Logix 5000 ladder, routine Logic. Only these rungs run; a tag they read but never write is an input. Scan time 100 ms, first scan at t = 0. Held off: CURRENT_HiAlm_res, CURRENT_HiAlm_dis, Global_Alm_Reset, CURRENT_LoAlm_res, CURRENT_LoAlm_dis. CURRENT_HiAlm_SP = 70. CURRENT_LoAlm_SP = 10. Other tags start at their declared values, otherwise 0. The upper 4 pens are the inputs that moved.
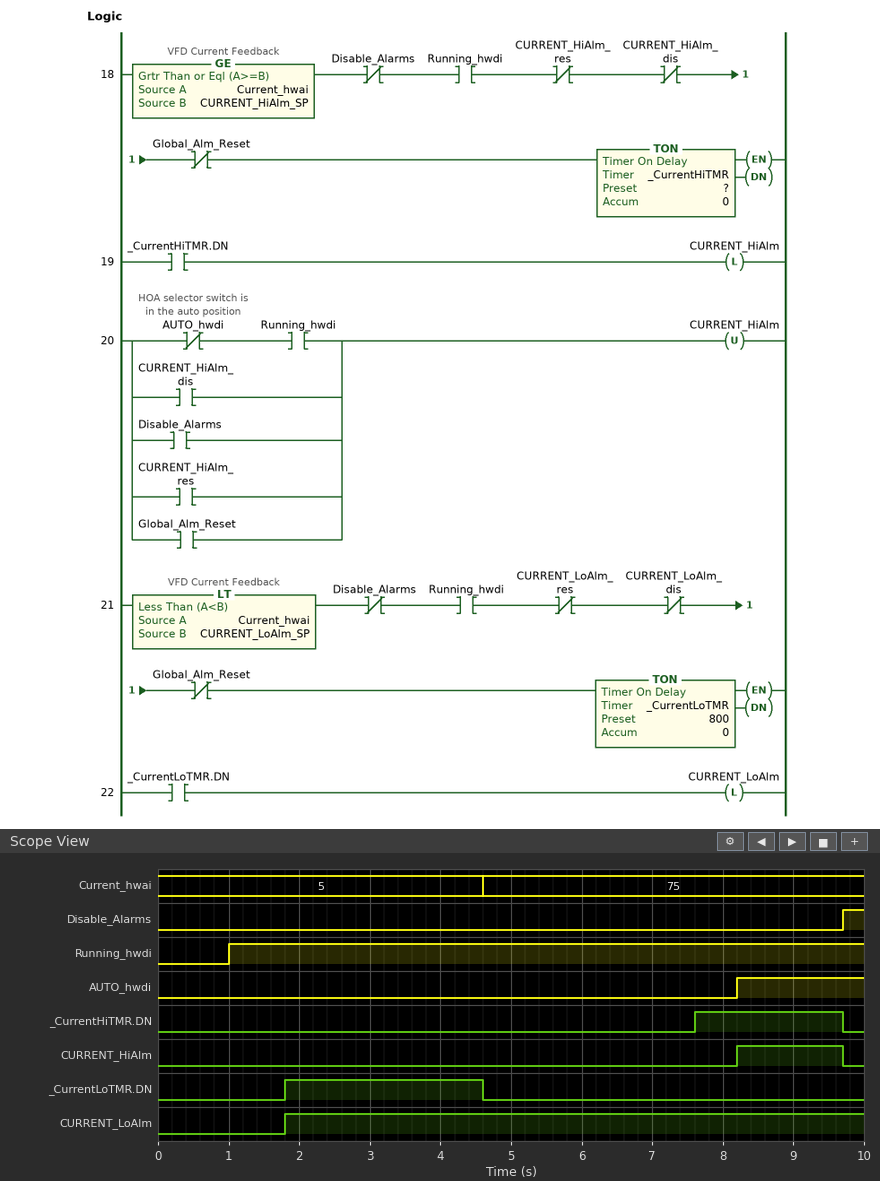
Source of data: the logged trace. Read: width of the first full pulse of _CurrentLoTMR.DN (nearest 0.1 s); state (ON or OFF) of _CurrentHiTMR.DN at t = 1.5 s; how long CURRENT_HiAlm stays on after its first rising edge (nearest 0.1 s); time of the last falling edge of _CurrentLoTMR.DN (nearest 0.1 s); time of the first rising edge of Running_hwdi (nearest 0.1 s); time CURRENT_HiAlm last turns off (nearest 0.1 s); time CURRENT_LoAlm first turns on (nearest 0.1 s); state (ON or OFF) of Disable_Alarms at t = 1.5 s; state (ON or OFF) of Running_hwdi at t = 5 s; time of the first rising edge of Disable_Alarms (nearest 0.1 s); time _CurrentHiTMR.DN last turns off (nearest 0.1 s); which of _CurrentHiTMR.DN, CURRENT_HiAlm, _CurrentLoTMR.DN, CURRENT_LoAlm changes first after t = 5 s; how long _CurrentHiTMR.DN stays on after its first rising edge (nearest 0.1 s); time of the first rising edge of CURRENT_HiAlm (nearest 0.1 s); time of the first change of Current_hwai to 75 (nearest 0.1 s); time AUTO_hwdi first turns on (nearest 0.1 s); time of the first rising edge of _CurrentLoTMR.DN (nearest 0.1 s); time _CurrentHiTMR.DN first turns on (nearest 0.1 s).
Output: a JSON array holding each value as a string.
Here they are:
["2.8 s", "OFF", "1.5 s", "4.6 s", "1.0 s", "9.7 s", "1.8 s", "OFF", "ON", "9.7 s", "9.7 s", "_CurrentHiTMR.DN", "2.1 s", "8.2 s", "4.6 s", "8.2 s", "1.8 s", "7.6 s"]
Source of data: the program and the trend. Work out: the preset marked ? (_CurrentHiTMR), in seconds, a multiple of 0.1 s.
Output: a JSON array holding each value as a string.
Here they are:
["3.0 s"]
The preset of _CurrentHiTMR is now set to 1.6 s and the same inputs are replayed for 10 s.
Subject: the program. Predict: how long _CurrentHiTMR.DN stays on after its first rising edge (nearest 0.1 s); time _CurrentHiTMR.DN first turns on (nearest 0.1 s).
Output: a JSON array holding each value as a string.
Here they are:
["3.5 s", "6.2 s"]
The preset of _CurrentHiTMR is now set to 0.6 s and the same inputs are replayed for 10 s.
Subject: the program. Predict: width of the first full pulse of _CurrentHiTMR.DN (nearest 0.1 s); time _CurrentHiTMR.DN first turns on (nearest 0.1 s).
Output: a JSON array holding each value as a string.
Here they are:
["4.5 s", "5.2 s"]
